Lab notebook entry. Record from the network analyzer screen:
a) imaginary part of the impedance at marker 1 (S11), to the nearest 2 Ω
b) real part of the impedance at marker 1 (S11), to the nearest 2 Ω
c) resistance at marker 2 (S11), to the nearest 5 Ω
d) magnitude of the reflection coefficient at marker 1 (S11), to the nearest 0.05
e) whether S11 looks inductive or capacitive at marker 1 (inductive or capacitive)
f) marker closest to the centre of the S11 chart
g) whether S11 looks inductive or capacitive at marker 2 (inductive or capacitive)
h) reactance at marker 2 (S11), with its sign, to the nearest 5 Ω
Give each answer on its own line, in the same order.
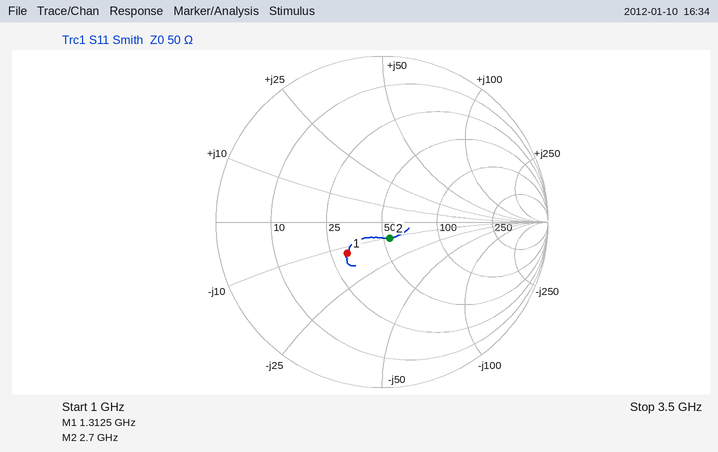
-12 Ω
30 Ω
55 Ω
0.30
capacitive
marker 2
capacitive
-10 Ω
